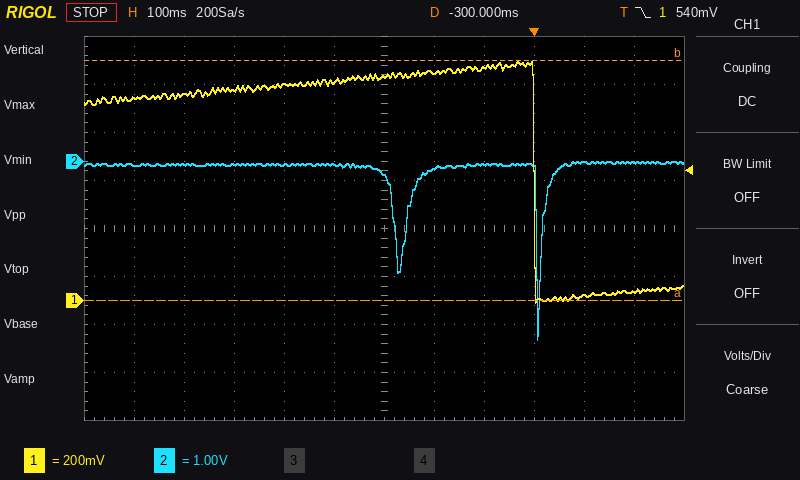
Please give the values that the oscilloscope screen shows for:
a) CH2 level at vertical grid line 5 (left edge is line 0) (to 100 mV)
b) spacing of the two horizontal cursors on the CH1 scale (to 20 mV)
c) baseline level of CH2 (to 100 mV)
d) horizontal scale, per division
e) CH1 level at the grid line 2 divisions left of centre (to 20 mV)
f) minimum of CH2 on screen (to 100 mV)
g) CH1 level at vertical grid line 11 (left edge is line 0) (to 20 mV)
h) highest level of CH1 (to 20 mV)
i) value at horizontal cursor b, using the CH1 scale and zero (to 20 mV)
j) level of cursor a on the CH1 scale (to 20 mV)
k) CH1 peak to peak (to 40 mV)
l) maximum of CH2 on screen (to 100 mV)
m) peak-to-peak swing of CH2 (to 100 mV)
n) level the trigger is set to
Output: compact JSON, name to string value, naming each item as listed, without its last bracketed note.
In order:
{"CH2 level at vertical grid line 5 (left edge is line 0)": "-100 mV", "spacing of the two horizontal cursors on the CH1 scale": "1.00 V", "baseline level of CH2": "-100 mV", "horizontal scale, per division": "100 ms", "CH1 level at the grid line 2 divisions left of centre": "900 mV", "minimum of CH2 on screen": "-3.7 V", "CH1 level at vertical grid line 11 (left edge is line 0)": "40 mV", "highest level of CH1": "1.00 V", "value at horizontal cursor b, using the CH1 scale and zero": "1.00 V", "level of cursor a on the CH1 scale": "0 mV", "CH1 peak to peak": "1.00 V", "maximum of CH2 on screen": "0.0 V", "peak-to-peak swing of CH2": "3.7 V", "level the trigger is set to": "540 mV"}
